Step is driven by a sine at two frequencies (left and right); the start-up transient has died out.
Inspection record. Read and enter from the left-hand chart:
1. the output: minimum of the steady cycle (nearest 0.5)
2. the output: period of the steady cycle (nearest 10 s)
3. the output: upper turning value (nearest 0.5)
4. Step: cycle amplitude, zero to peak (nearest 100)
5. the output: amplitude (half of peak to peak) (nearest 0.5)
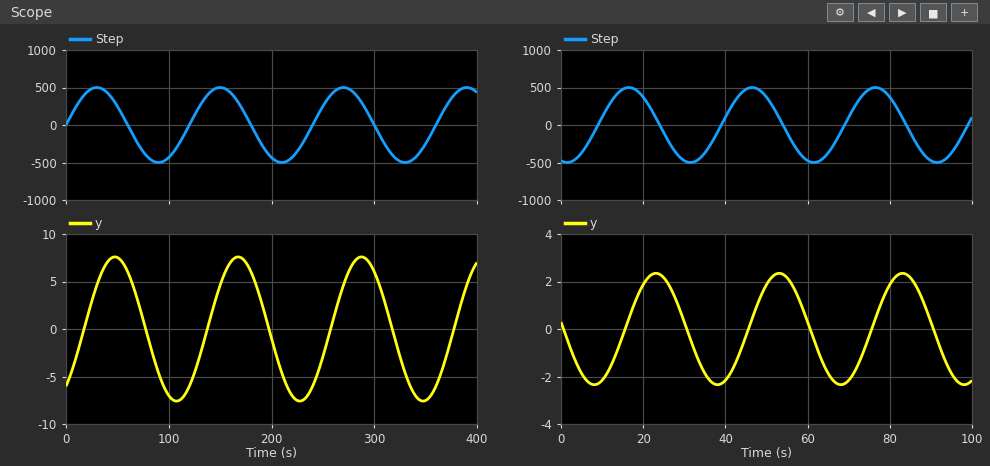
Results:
-7.5
120 s
7.5
500
7.5
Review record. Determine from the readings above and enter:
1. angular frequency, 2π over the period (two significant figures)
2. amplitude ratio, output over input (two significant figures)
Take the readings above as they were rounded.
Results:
0.052 rad/s
0.015
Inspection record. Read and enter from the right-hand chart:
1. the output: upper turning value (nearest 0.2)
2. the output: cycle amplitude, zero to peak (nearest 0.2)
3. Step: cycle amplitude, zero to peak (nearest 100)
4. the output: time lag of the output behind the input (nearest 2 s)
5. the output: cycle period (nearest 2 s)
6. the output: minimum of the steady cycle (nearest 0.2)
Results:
2.4
2.4
500
6 s
30 s
-2.4
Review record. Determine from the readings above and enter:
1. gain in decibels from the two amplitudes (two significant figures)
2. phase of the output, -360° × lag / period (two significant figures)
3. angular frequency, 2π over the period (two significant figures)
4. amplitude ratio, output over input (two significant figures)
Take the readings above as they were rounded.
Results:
-46 dB
-72°
0.21 rad/s
0.0048
